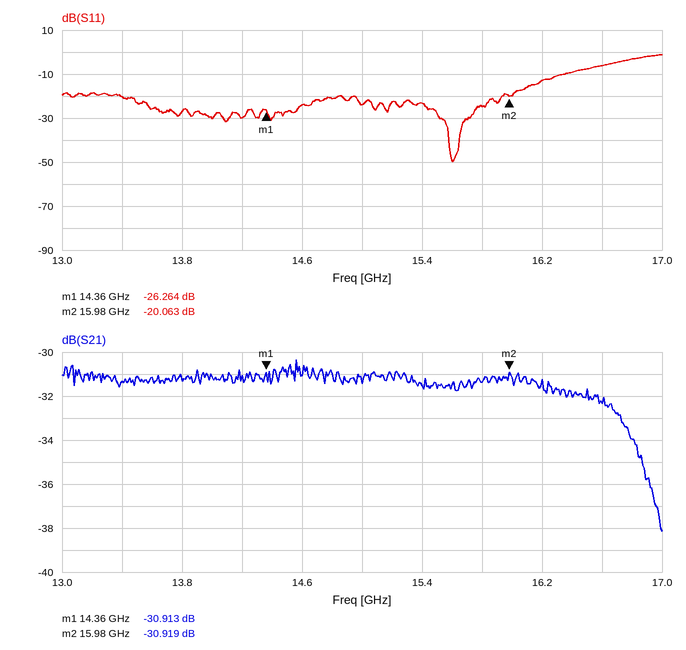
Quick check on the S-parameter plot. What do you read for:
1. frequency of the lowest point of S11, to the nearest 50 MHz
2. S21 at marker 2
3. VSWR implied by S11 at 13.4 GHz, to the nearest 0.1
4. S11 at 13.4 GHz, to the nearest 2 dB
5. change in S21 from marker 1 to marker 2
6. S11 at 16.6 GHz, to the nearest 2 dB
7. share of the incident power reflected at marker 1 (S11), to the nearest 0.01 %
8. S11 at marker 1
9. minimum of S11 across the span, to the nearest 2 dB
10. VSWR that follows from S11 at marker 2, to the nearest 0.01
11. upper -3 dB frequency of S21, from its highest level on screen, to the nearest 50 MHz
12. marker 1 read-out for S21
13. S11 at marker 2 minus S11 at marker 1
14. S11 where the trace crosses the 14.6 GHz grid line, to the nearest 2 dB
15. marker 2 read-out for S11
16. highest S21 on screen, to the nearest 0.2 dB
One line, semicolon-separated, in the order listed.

15.60 GHz; -30.919 dB; 1.2; -20 dB; -0.006 dB; -6 dB; 0.24 %; -26.264 dB; -50 dB; 1.22; 16.75 GHz; -30.913 dB; 6.201 dB; -24 dB; -20.063 dB; -30.4 dB
